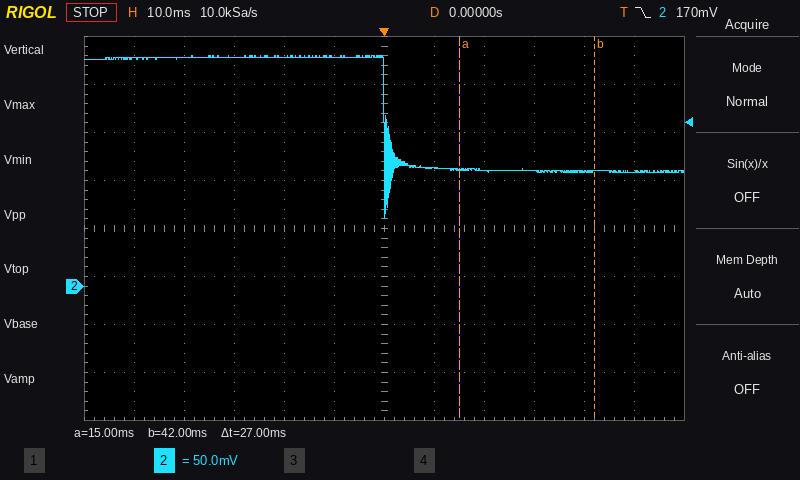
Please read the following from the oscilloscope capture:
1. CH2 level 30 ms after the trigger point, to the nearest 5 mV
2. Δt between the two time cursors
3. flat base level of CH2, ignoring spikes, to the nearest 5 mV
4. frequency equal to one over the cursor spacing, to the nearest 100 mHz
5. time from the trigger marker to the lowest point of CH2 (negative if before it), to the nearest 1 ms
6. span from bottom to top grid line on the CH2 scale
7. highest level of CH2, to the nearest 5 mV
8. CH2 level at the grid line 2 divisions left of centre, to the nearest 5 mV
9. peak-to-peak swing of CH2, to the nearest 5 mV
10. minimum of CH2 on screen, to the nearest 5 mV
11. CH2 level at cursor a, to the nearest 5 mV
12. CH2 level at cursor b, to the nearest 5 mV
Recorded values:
120 mV
27 ms
120 mV
37.0 Hz
0 ms
400 mV
240 mV
240 mV
170 mV
70 mV
120 mV
120 mV
